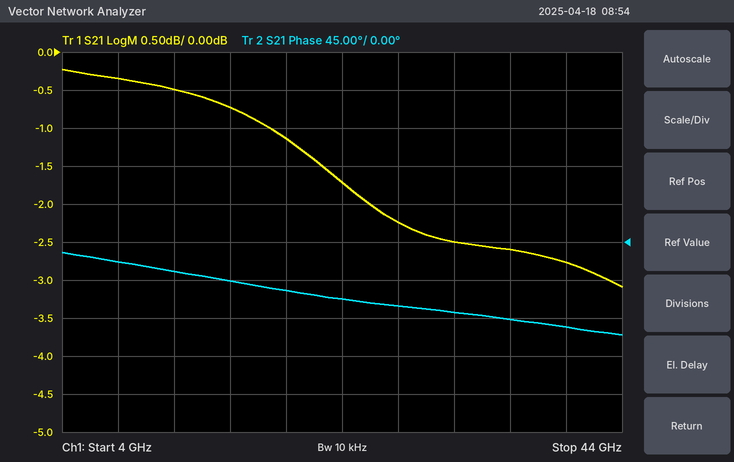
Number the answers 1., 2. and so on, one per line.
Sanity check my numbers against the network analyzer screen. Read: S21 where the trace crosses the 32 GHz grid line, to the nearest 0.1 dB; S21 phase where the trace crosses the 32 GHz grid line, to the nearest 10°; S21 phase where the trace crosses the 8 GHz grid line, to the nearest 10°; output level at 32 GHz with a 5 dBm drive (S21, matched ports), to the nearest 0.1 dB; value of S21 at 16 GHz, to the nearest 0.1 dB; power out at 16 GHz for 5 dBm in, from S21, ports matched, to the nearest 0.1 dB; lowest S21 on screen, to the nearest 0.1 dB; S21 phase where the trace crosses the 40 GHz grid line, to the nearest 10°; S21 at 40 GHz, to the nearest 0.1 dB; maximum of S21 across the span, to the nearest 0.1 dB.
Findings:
1. -2.5 dB
2. -80°
3. -20°
4. 2.5 dBm
5. -0.7 dB
6. 4.3 dBm
7. -3.1 dB
8. -100°
9. -2.8 dB
10. -0.2 dB
